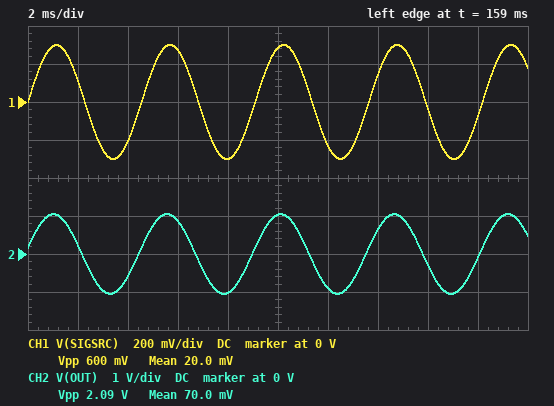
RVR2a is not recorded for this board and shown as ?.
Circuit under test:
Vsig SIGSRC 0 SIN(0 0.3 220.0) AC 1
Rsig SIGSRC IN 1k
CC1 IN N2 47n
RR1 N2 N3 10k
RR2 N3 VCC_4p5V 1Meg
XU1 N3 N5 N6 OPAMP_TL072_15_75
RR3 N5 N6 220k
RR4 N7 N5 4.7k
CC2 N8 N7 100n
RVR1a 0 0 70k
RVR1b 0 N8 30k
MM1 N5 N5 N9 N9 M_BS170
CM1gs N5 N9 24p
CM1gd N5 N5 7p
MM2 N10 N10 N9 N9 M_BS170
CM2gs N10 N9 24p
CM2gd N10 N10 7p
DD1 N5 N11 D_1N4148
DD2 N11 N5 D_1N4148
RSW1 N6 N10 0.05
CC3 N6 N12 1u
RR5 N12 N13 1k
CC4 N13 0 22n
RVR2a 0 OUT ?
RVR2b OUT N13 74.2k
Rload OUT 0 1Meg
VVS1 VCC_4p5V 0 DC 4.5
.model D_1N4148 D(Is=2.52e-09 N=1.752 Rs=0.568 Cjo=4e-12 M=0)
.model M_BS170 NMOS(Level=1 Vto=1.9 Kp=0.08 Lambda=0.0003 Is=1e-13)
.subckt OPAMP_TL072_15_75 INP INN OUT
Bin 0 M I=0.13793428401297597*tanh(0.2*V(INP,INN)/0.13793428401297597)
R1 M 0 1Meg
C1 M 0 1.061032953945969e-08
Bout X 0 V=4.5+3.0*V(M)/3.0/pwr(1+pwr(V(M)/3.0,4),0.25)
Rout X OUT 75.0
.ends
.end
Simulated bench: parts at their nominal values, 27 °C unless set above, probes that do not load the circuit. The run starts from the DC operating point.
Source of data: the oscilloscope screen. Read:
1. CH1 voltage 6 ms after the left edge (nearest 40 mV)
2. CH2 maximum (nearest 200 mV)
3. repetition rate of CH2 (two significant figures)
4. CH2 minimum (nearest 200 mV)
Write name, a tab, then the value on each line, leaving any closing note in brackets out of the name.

CH1 voltage 6 ms after the left edge	280 mV
CH2 maximum	1.0 V
repetition rate of CH2	220 Hz
CH2 minimum	-1.0 V
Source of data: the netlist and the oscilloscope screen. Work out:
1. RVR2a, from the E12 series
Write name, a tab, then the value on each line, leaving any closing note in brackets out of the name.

RVR2a, from the E12 series	82 kΩ
